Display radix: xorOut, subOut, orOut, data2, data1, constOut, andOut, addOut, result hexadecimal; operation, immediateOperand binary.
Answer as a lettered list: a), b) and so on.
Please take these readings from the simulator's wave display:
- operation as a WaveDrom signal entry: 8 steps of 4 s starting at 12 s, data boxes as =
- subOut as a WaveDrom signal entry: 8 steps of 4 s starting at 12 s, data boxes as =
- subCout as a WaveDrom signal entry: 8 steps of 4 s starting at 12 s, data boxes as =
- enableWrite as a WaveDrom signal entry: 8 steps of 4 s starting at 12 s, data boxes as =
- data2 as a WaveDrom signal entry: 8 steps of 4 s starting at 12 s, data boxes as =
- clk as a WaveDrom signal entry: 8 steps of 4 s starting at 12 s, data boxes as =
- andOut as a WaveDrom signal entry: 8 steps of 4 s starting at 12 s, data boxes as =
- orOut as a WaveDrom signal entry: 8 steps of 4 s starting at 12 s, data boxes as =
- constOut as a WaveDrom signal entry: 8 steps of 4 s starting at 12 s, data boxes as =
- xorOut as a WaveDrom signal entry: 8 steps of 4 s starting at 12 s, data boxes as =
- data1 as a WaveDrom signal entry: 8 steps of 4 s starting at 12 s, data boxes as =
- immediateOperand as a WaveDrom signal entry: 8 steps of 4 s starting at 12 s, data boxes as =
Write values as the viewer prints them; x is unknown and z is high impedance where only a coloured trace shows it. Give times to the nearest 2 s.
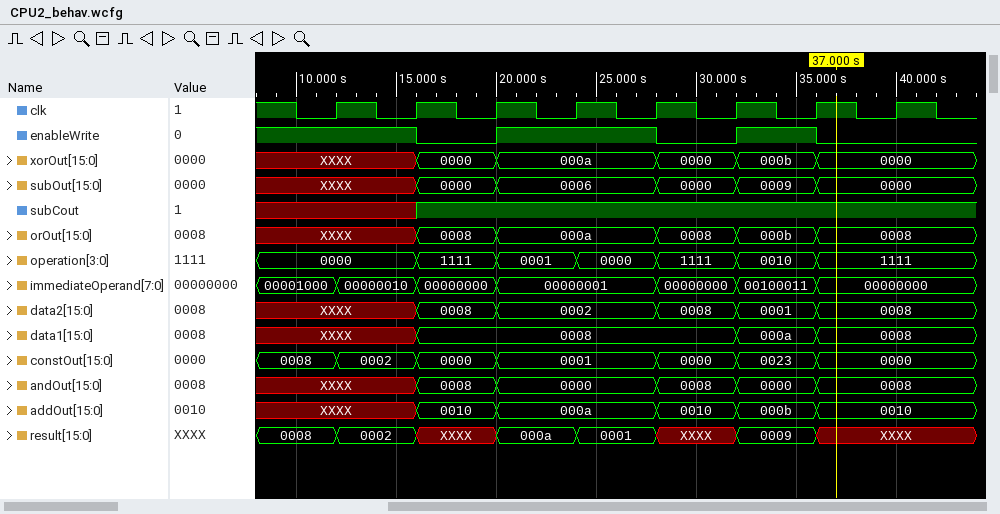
a) {name: 'operation', wave: '=======.', data: '0000 1111 0001 0000 1111 0010 1111'}
b) {name: 'subOut', wave: 'x==.===.', data: '0000 0006 0000 0009 0000'}
c) {name: 'subCout', wave: 'x1......'}
d) {name: 'enableWrite', wave: '101.010.'}
e) {name: 'data2', wave: 'x==.===.', data: '0008 0002 0008 0001 0008'}
f) {name: 'clk', wave: 'p.......'}
g) {name: 'andOut', wave: 'x==.===.', data: '0008 0000 0008 0000 0008'}
h) {name: 'orOut', wave: 'x==.===.', data: '0008 000a 0008 000b 0008'}
i) {name: 'constOut', wave: '===.===.', data: '0002 0000 0001 0000 0023 0000'}
j) {name: 'xorOut', wave: 'x==.===.', data: '0000 000a 0000 000b 0000'}
k) {name: 'data1', wave: 'x=...==.', data: '0008 000a 0008'}
l) {name: 'immediateOperand', wave: '===.===.', data: '00000010 00000000 00000001 00000000 00100011 00000000'}
